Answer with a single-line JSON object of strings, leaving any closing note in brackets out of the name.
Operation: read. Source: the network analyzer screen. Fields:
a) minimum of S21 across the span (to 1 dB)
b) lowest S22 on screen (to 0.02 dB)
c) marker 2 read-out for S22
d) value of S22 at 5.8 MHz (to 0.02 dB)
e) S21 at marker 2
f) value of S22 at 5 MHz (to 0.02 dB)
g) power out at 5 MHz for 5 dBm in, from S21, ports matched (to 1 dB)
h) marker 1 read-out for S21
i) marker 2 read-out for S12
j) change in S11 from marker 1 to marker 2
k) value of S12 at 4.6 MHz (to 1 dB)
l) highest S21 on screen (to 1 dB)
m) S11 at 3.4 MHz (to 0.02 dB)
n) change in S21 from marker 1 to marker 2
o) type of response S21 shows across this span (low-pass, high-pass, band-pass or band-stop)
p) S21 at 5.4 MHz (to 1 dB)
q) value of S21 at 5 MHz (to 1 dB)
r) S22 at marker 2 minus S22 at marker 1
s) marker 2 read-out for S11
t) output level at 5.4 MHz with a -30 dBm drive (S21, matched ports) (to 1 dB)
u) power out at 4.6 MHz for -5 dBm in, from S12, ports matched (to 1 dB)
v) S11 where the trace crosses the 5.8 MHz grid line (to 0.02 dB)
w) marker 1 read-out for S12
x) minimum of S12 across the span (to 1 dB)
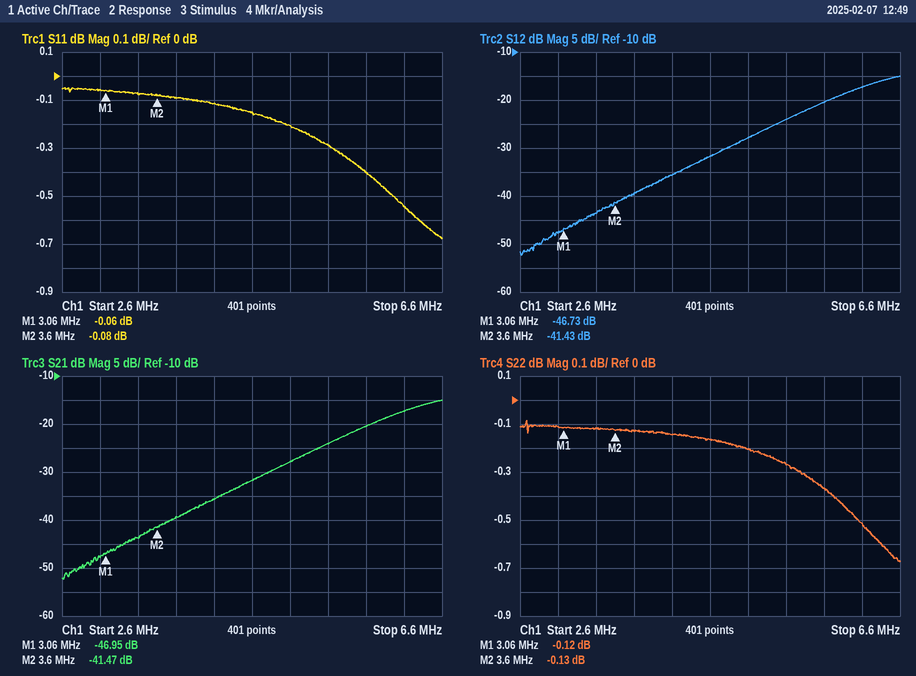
{"minimum of S21 across the span": "-52 dB", "lowest S22 on screen": "-0.68 dB", "marker 2 read-out for S22": "-0.13 dB", "value of S22 at 5.8 MHz": "-0.36 dB", "S21 at marker 2": "-41.47 dB", "value of S22 at 5 MHz": "-0.20 dB", "power out at 5 MHz for 5 dBm in, from S21, ports matched": "-23 dBm", "marker 1 read-out for S21": "-46.95 dB", "marker 2 read-out for S12": "-41.43 dB", "change in S11 from marker 1 to marker 2": "-0.02 dB", "value of S12 at 4.6 MHz": "-32 dB", "highest S21 on screen": "-15 dB", "S11 at 3.4 MHz": "-0.08 dB", "change in S21 from marker 1 to marker 2": "5.48 dB", "type of response S21 shows across this span": "high-pass", "S21 at 5.4 MHz": "-24 dB", "value of S21 at 5 MHz": "-28 dB", "S22 at marker 2 minus S22 at marker 1": "-0.01 dB", "marker 2 read-out for S11": "-0.08 dB", "output level at 5.4 MHz with a -30 dBm drive (S21, matched ports)": "-54 dBm", "power out at 4.6 MHz for -5 dBm in, from S12, ports matched": "-37 dBm", "S11 where the trace crosses the 5.8 MHz grid line": "-0.40 dB", "marker 1 read-out for S12": "-46.73 dB", "minimum of S12 across the span": "-52 dB"}
